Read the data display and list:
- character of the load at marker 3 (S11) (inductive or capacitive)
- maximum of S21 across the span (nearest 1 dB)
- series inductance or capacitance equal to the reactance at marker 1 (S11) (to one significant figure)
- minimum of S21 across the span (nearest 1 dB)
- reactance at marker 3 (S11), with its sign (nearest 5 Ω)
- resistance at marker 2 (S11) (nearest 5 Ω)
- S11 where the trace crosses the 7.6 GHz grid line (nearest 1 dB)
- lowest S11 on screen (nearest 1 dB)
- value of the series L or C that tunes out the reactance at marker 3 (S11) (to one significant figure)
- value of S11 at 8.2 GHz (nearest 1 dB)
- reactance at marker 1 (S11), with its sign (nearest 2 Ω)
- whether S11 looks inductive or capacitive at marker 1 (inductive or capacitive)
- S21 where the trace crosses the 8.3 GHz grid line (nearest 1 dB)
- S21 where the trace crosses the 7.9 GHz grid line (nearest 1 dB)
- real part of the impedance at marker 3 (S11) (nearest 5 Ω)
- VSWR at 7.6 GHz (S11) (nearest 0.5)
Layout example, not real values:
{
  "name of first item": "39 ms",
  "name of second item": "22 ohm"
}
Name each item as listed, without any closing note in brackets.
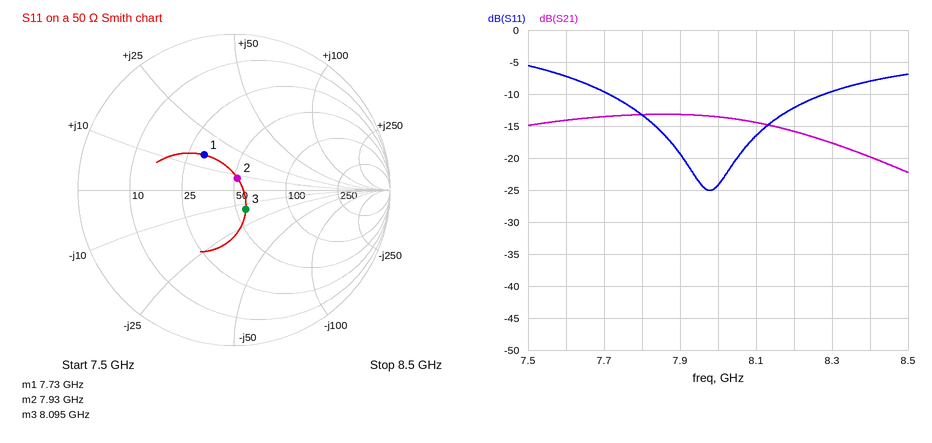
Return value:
{
  "character of the load at marker 3 (S11)": "capacitive",
  "maximum of S21 across the span": "-13 dB",
  "series inductance or capacitance equal to the reactance at marker 1 (S11)": "300 pH",
  "minimum of S21 across the span": "-22 dB",
  "reactance at marker 3 (S11), with its sign": "-15 Ω",
  "resistance at marker 2 (S11)": "50 Ω",
  "S11 where the trace crosses the 7.6 GHz grid line": "-7 dB",
  "lowest S11 on screen": "-25 dB",
  "value of the series L or C that tunes out the reactance at marker 3 (S11)": "300 pH",
  "value of S11 at 8.2 GHz": "-12 dB",
  "reactance at marker 1 (S11), with its sign": "+16 Ω",
  "whether S11 looks inductive or capacitive at marker 1": "inductive",
  "S21 where the trace crosses the 8.3 GHz grid line": "-18 dB",
  "S21 where the trace crosses the 7.9 GHz grid line": "-13 dB",
  "real part of the impedance at marker 3 (S11)": "55 Ω",
  "VSWR at 7.6 GHz (S11)": "2.5"
}
